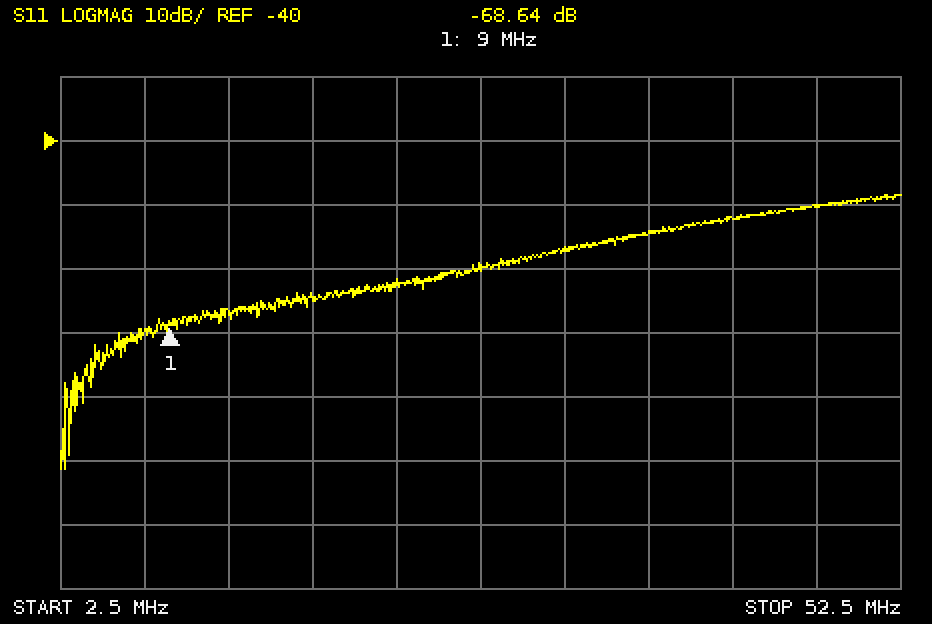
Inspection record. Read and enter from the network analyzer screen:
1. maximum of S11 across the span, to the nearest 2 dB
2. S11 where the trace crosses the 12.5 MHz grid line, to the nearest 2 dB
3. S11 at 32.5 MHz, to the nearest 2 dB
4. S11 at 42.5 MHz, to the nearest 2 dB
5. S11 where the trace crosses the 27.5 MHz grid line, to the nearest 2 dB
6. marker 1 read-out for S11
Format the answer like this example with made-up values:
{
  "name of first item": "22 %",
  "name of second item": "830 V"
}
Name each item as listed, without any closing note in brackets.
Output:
{
  "maximum of S11 across the span, to the nearest 2 dB": "-48 dB",
  "S11 where the trace crosses the 12.5 MHz grid line, to the nearest 2 dB": "-66 dB",
  "S11 at 32.5 MHz, to the nearest 2 dB": "-56 dB",
  "S11 at 42.5 MHz, to the nearest 2 dB": "-52 dB",
  "S11 where the trace crosses the 27.5 MHz grid line, to the nearest 2 dB": "-60 dB",
  "marker 1 read-out for S11": "-68.64 dB"
}
